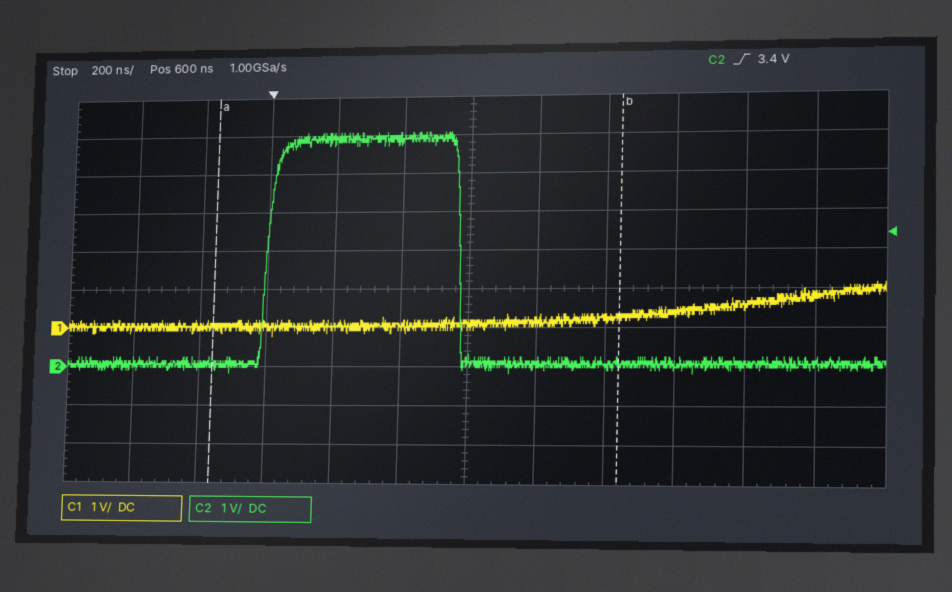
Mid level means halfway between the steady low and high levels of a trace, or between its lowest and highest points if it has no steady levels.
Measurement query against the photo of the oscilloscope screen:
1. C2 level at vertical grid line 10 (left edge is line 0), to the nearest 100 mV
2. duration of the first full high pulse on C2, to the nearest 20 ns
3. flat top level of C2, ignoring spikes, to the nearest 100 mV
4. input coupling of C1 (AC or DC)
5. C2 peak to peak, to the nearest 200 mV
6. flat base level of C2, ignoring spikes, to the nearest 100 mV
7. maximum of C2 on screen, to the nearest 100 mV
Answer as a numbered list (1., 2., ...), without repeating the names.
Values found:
1. 100 mV
2. 580 ns
3. 5.9 V
4. DC
5. 6.2 V
6. 100 mV
7. 6.1 V
